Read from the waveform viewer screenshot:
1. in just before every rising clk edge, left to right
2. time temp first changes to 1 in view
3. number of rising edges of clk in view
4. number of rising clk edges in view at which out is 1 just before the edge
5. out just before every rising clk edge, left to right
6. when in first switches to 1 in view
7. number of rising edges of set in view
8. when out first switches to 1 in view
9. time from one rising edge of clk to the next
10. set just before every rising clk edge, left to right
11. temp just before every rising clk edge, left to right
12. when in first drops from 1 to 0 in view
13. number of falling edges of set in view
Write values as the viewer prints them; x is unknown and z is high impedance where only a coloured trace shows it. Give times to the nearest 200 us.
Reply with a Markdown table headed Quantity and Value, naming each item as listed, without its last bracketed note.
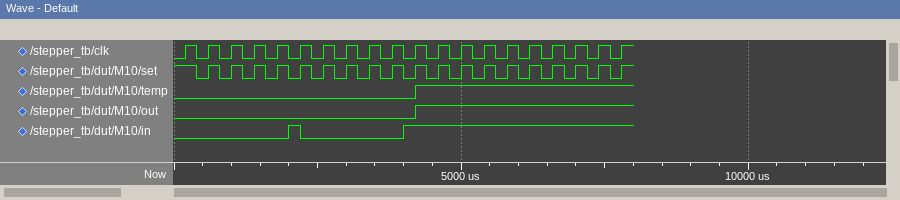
| Quantity | Value |
|---|---|
| in just before every rising clk edge, left to right | 0 0 0 0 0 1 0 0 0 0 1 1 1 1 1 1 1 1 1 1 |
| time temp first changes to 1 in view | 4200 us |
| number of rising edges of clk in view | 20 |
| number of rising clk edges in view at which out is 1 just before the edge | 9 |
| out just before every rising clk edge, left to right | 0 0 0 0 0 0 0 0 0 0 0 1 1 1 1 1 1 1 1 1 |
| when in first switches to 1 in view | 2000 us |
| number of rising edges of set in view | 19 |
| when out first switches to 1 in view | 4200 us |
| time from one rising edge of clk to the next | 400 us |
| set just before every rising clk edge, left to right | 1 0 0 0 0 0 0 0 0 0 0 0 0 0 0 0 0 0 0 0 |
| temp just before every rising clk edge, left to right | 0 0 0 0 0 0 0 0 0 0 0 1 1 1 1 1 1 1 1 1 |
| when in first drops from 1 to 0 in view | 2200 us |
| number of falling edges of set in view | 19 |
